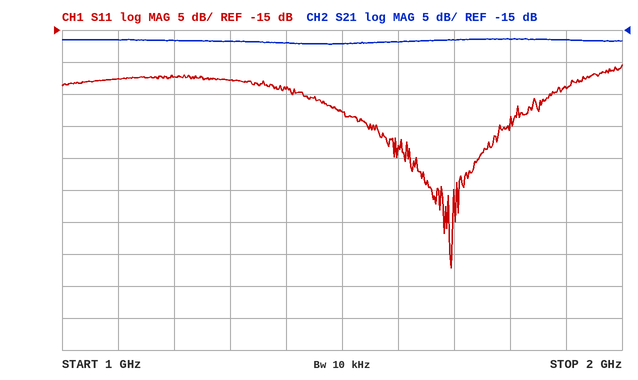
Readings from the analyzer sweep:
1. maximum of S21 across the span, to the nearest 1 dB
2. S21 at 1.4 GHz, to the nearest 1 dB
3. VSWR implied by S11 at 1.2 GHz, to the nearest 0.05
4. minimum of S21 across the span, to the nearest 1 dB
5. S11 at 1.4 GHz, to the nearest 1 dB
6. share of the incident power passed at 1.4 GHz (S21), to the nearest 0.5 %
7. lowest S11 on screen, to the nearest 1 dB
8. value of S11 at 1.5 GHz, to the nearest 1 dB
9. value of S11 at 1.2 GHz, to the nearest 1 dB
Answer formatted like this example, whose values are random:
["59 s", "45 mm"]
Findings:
["-16 dB", "-17 dB", "1.15", "-17 dB", "-24 dB", "2.0 %", "-52 dB", "-28 dB", "-22 dB"]
